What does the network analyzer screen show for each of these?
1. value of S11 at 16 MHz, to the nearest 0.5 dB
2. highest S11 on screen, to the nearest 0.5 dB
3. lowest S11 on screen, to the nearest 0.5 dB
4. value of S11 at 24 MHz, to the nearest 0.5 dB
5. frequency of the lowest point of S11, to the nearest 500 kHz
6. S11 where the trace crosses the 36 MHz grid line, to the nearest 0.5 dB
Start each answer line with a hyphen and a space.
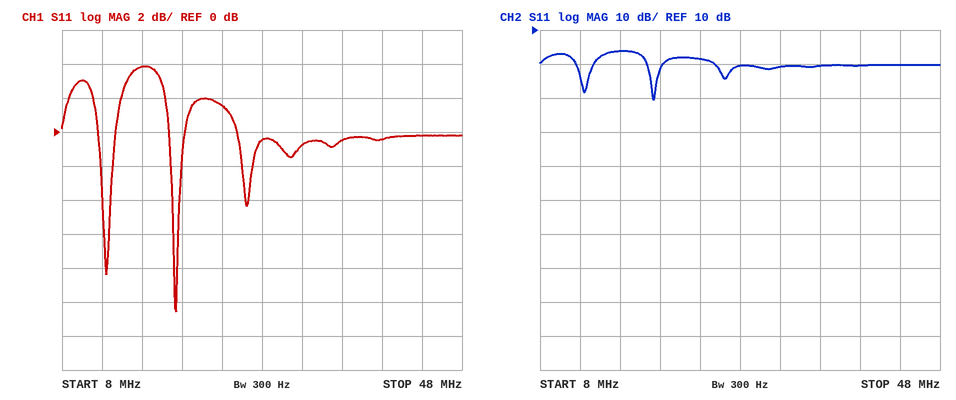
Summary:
- 4.0 dB
- 4.0 dB
- -10.5 dB
- 1.5 dB
- 19.5 MHz
- -0.5 dB
